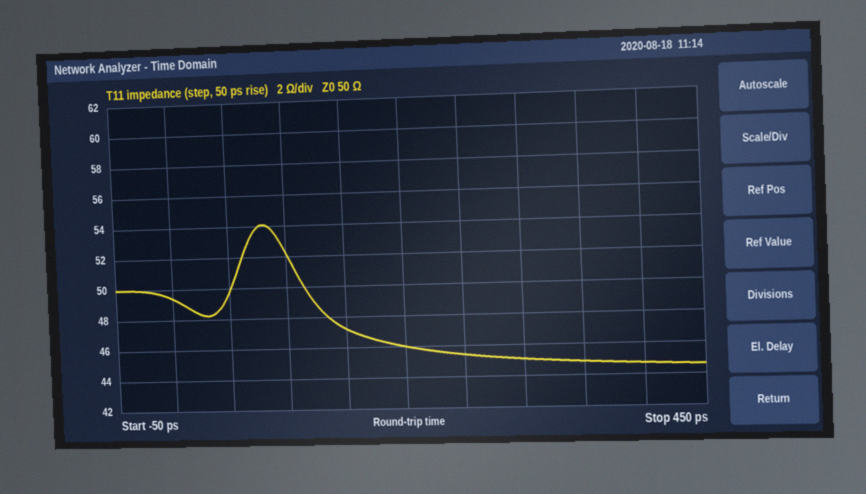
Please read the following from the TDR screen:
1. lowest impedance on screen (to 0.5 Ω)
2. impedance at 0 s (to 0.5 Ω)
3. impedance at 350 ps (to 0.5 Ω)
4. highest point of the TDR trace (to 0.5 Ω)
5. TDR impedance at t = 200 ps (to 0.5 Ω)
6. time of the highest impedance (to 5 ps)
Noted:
44.5 Ω
49.5 Ω
45.0 Ω
54.0 Ω
46.0 Ω
80 ps
